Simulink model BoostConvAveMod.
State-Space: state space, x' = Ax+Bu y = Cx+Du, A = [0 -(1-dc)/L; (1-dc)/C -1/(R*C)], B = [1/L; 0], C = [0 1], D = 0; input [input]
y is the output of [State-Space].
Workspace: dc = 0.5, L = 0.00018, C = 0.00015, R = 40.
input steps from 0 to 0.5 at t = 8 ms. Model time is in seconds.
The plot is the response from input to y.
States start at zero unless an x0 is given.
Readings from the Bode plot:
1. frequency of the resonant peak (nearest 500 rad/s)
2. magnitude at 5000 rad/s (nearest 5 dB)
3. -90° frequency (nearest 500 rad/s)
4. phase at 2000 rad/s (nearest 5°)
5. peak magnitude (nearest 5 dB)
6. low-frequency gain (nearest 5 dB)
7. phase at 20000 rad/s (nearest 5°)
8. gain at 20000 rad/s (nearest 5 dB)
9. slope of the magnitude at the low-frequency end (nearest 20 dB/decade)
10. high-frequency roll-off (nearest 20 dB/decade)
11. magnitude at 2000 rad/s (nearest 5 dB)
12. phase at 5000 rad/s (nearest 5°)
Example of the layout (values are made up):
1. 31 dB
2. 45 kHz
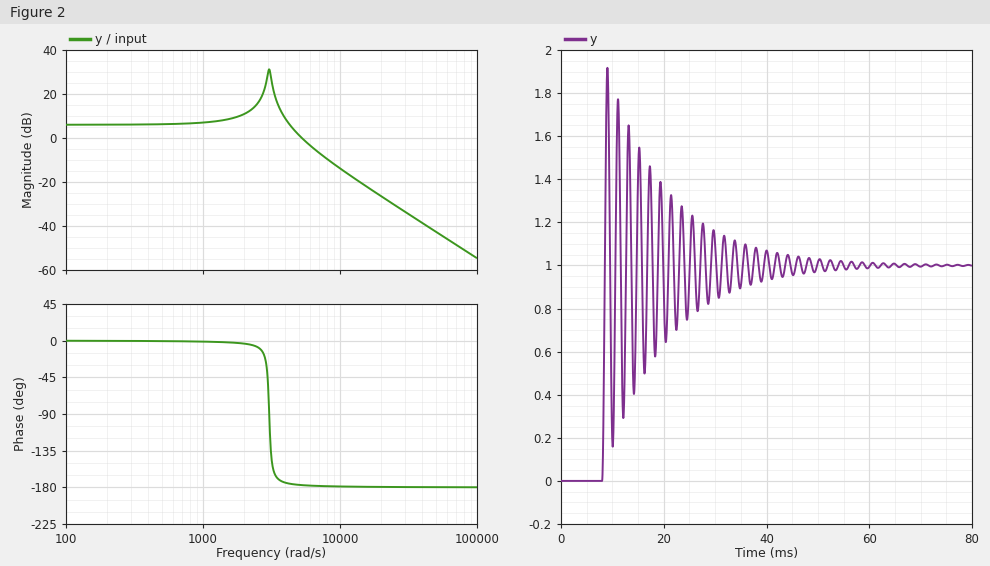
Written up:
1. 3000 rad/s
2. 0 dB
3. 3000 rad/s
4. -5°
5. 30 dB
6. 5 dB
7. -180°
8. -25 dB
9. 0 dB/decade
10. -40 dB/decade
11. 10 dB
12. -175°
